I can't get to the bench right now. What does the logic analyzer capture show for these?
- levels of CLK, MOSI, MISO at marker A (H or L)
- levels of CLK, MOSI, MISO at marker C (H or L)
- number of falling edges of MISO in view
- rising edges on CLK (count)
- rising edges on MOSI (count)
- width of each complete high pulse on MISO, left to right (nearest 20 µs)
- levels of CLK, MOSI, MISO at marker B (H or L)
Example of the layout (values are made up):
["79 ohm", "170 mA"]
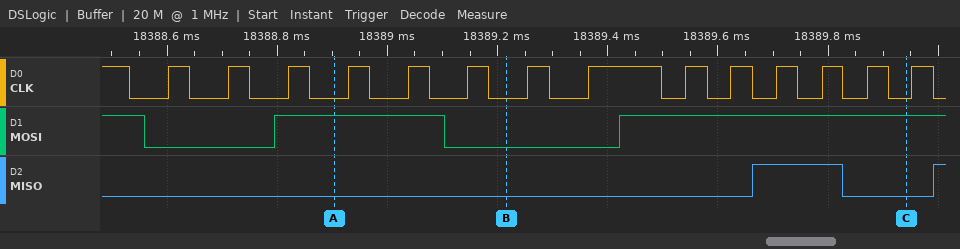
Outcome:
["CLK=L, MOSI=H, MISO=L", "CLK=L, MOSI=H, MISO=L", "1", "14", "2", "160 µs", "CLK=L, MOSI=L, MISO=L"]
